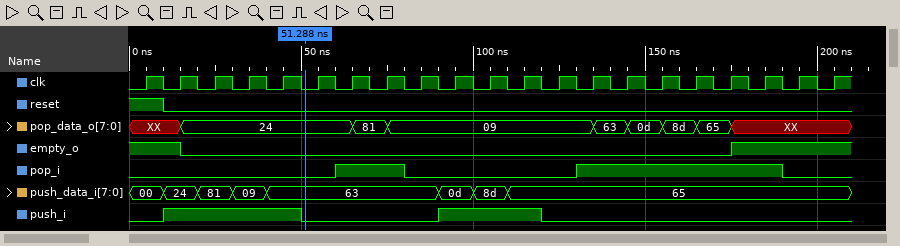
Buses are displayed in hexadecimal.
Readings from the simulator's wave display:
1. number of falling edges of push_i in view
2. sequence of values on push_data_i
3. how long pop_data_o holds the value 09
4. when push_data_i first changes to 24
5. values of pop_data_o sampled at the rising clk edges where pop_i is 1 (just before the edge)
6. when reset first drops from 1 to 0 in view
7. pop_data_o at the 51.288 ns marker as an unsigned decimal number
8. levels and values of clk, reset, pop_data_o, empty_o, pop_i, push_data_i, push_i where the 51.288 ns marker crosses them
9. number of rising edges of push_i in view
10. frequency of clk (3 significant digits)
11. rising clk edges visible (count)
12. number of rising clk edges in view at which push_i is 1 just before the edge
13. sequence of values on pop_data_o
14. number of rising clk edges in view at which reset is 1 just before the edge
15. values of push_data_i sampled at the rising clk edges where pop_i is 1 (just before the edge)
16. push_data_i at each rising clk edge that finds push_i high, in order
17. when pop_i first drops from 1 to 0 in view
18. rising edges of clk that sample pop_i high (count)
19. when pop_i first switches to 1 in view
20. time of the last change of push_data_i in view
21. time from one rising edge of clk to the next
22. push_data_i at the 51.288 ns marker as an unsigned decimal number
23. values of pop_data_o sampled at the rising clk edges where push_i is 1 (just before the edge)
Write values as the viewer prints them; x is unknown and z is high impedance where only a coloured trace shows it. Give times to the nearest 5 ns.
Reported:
2
00, 24, 81, 09, 63, 0d, 8d, 65
60 ns
10 ns
24, 81, 09, 63, 0d, 8d, 65, XX
10 ns
36
clk=0, reset=0, pop_data_o=24, empty_o=0, pop_i=0, push_data_i=63, push_i=0
2
100 MHz
21
7
XX, 24, 81, 09, 63, 0d, 8d, 65, XX
1
63, 63, 65, 65, 65, 65, 65, 65
24, 81, 09, 63, 0d, 8d, 65
80 ns
8
60 ns
110 ns
10 ns
99
XX, 24, 24, 24, 09, 09, 09
